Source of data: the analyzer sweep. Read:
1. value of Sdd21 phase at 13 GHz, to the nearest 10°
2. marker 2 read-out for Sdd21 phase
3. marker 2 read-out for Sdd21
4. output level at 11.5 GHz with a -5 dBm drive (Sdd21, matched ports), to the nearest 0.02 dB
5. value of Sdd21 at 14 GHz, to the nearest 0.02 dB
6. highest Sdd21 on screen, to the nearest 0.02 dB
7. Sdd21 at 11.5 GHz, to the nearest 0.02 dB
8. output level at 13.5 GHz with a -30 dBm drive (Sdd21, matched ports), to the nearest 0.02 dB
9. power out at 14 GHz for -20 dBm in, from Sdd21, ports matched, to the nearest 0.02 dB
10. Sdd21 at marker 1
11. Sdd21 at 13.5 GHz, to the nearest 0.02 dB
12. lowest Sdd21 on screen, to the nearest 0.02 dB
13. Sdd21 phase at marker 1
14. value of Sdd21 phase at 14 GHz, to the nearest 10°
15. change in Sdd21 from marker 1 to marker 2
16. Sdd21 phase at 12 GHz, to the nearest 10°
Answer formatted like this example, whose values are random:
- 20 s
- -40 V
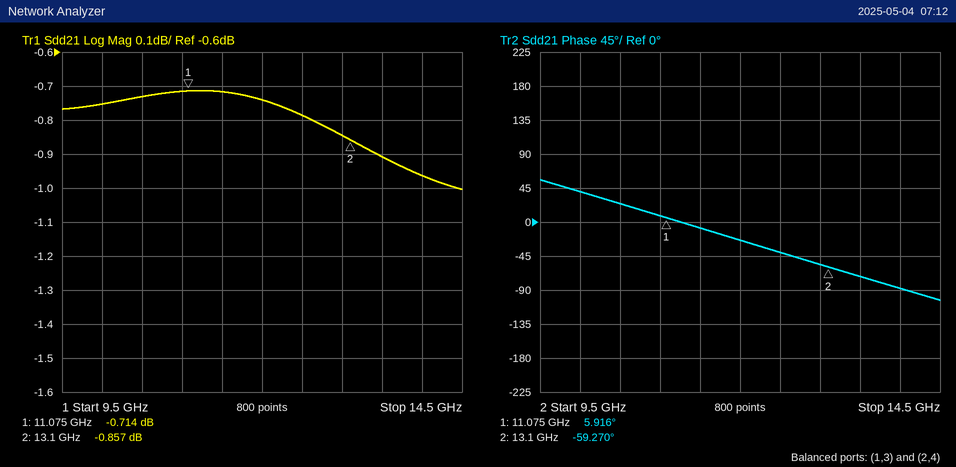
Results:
- -60°
- -59.270°
- -0.857 dB
- -5.72 dBm
- -0.96 dB
- -0.72 dB
- -0.72 dB
- -30.90 dBm
- -20.96 dBm
- -0.714 dB
- -0.90 dB
- -1.00 dB
- 5.916°
- -90°
- -0.143 dB
- -20°
